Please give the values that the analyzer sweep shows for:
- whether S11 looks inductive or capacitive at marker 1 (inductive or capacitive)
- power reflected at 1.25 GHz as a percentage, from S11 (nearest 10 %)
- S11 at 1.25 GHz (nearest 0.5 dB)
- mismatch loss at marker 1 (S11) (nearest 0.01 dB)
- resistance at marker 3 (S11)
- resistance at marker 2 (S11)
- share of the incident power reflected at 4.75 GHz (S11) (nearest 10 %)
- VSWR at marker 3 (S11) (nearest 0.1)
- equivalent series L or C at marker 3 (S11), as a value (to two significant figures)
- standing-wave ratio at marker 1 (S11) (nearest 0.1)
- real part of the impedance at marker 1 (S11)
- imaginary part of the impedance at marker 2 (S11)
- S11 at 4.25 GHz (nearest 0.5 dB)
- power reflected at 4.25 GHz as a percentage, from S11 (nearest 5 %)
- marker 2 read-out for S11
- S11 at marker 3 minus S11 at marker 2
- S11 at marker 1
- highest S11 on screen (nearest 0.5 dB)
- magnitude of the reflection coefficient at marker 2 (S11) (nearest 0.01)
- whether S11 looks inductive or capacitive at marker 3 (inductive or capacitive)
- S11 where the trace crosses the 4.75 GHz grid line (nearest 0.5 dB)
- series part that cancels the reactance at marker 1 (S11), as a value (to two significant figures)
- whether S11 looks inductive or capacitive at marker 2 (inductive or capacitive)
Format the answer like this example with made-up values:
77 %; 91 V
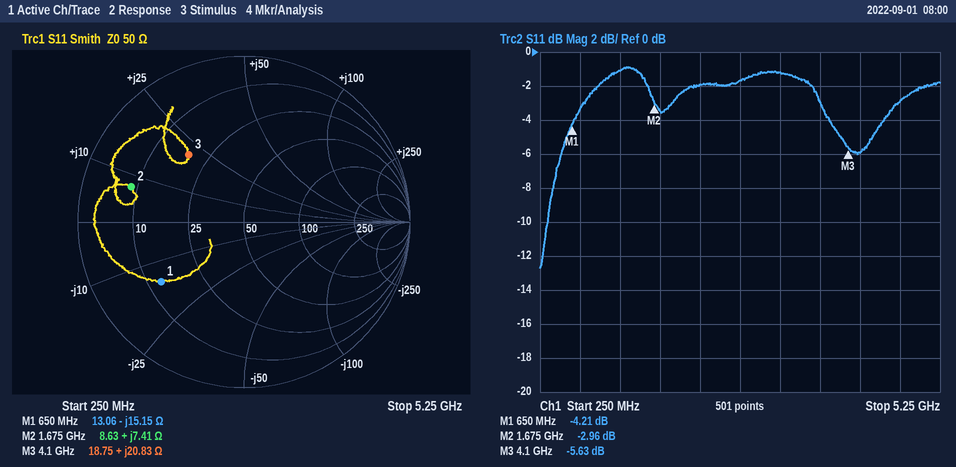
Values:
capacitive; 80 %; -1.0 dB; 2.07 dB; 18.75 Ω; 8.63 Ω; 50 %; 3.2; 810 pH; 4.2; 13.06 Ω; +7.41 Ω; -6.0 dB; 25 %; -2.96 dB; -2.67 dB; -4.21 dB; -1.0 dB; 0.71; inductive; -3.0 dB; 3.7 nH; inductive
